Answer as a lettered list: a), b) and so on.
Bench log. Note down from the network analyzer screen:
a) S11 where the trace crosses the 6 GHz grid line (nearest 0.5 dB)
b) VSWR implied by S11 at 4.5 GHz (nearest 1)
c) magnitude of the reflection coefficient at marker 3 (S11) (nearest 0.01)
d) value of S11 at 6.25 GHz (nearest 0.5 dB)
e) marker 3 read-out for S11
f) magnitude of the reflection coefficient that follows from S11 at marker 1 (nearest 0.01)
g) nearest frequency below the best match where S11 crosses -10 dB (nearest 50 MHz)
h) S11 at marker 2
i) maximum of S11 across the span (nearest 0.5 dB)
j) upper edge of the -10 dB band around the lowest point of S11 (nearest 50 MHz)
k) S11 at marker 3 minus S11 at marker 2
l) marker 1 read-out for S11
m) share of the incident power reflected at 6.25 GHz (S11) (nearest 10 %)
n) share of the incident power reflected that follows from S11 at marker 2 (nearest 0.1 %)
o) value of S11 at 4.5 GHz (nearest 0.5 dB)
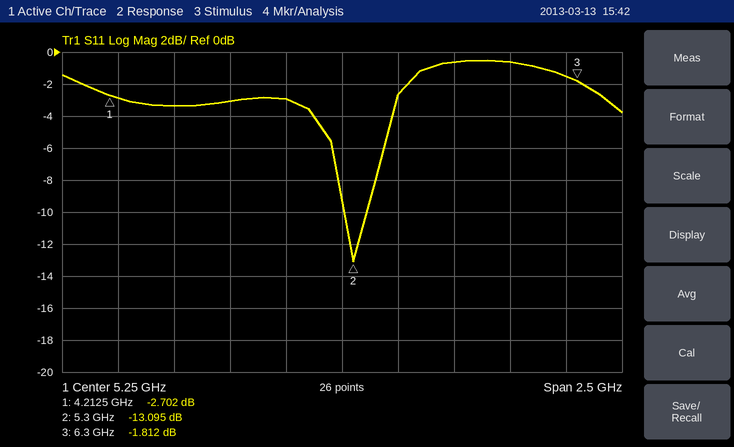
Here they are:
a) -0.5 dB
b) 5
c) 0.81
d) -1.5 dB
e) -1.812 dB
f) 0.73
g) 5.25 GHz
h) -13.095 dB
i) -0.5 dB
j) 5.35 GHz
k) 11.283 dB
l) -2.702 dB
m) 70 %
n) 4.9 %
o) -3.5 dB
